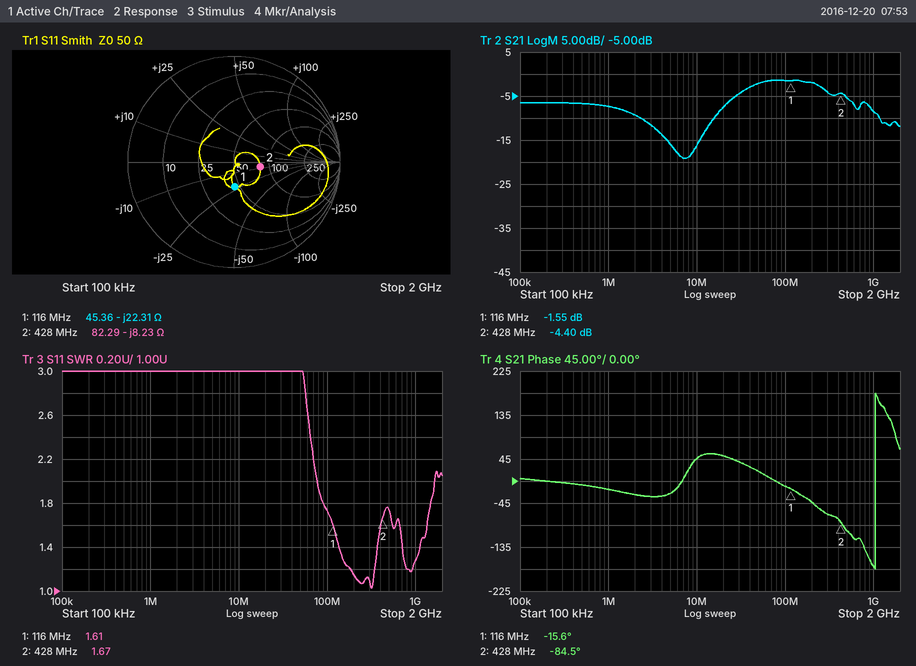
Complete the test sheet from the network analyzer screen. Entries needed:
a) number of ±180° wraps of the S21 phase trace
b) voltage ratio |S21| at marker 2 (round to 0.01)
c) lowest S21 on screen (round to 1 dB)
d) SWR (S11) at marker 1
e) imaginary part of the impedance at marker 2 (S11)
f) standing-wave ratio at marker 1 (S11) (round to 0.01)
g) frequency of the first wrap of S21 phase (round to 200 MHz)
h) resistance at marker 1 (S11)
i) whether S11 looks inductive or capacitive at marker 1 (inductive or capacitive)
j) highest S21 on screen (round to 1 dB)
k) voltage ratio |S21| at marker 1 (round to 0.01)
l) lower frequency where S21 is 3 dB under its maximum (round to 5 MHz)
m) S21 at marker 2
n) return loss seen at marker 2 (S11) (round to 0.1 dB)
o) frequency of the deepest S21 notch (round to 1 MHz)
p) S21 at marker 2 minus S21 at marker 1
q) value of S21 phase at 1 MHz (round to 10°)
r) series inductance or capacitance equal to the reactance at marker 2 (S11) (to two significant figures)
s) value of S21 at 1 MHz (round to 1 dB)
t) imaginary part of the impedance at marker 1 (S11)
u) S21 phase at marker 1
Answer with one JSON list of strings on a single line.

["1", "0.60", "-19 dB", "1.61", "-8.23 Ω", "1.61", "1.0 GHz", "45.36 Ω", "capacitive", "-1 dB", "0.84", "30 MHz", "-4.40 dB", "12.0 dB", "7 MHz", "-2.85 dB", "-20°", "45 pF", "-7 dB", "-22.31 Ω", "-15.6°"]
